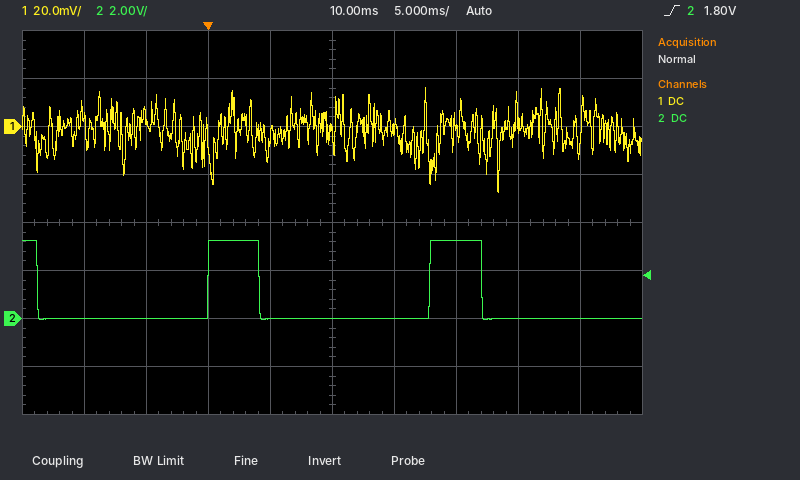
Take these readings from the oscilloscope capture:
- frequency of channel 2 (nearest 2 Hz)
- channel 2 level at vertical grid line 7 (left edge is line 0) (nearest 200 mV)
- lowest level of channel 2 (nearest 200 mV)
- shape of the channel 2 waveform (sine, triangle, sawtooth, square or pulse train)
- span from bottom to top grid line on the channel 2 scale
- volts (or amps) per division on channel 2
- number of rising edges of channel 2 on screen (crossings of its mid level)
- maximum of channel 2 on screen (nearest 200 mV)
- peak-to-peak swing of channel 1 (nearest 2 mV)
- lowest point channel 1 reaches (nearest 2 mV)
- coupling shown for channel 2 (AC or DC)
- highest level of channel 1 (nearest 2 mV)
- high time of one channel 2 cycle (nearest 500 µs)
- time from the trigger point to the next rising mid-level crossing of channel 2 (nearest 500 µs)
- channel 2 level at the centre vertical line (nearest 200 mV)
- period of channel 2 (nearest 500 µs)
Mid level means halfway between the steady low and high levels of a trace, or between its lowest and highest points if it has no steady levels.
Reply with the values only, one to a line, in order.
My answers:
56 Hz
3.2 V
0.0 V
pulse train
16 V
2 V
2
3.2 V
44 mV
-28 mV
DC
16 mV
4.0 ms
18.0 ms
0.0 V
18.0 ms
